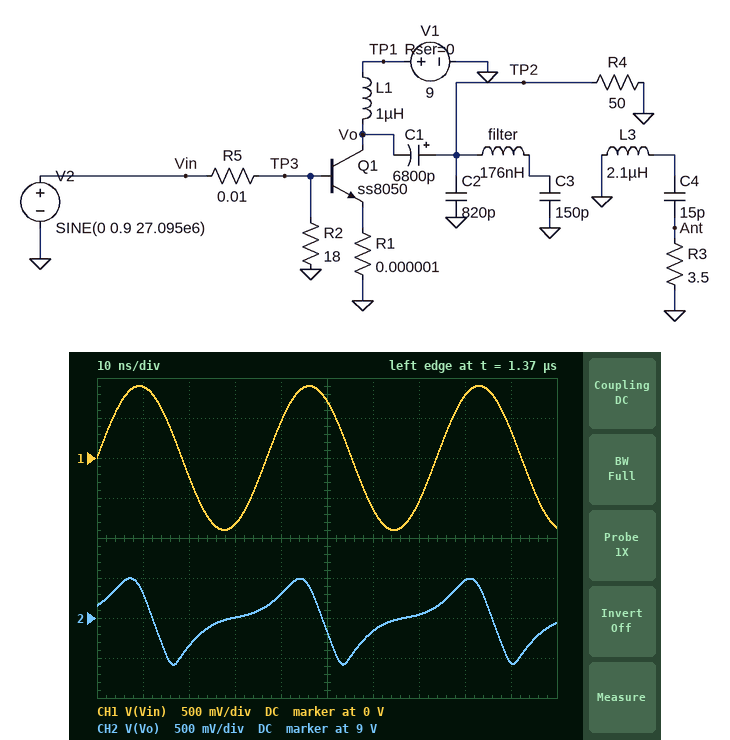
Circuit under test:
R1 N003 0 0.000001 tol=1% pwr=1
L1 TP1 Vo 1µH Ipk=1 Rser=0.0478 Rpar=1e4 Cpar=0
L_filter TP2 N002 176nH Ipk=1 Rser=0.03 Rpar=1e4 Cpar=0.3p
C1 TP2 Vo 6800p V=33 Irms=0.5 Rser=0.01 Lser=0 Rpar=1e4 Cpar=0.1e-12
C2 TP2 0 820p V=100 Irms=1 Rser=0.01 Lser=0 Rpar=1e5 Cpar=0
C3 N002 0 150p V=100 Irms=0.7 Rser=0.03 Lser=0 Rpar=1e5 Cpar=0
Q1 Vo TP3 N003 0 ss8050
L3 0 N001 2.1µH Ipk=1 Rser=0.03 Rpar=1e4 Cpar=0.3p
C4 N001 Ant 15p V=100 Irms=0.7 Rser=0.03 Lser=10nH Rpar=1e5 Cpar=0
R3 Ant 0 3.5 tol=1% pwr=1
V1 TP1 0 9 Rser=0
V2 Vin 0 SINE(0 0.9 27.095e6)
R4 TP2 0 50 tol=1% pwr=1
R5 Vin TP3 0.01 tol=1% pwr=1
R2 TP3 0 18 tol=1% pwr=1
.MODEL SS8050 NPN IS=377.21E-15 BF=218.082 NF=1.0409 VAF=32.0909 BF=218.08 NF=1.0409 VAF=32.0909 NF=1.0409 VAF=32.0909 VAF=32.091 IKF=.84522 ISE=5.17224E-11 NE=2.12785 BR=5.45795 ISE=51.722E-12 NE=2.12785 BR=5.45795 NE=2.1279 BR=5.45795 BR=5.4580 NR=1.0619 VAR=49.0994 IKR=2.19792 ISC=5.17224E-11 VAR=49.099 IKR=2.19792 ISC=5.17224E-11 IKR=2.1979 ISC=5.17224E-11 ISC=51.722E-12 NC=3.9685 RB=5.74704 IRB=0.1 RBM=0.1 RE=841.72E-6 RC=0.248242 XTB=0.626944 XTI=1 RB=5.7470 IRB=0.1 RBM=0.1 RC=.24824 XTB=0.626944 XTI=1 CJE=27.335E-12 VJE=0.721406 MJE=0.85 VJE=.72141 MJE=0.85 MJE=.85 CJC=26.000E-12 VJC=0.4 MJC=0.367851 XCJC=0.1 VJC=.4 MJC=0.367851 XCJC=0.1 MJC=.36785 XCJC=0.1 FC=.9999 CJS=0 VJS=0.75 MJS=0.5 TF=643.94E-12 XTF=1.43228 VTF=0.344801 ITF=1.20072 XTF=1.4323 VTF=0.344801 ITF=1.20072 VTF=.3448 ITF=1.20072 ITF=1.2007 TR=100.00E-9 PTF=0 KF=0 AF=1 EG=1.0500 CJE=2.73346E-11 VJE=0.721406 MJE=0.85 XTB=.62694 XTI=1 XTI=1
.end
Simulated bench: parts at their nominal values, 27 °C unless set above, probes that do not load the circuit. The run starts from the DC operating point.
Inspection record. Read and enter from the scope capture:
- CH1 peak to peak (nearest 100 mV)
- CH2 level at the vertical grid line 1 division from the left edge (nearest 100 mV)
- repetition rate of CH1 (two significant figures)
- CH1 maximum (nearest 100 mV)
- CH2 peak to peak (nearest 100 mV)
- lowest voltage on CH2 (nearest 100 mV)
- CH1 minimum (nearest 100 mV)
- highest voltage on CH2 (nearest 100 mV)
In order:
1.8 V
9.3 V
27 MHz
900 mV
1.1 V
8.4 V
-900 mV
9.5 V
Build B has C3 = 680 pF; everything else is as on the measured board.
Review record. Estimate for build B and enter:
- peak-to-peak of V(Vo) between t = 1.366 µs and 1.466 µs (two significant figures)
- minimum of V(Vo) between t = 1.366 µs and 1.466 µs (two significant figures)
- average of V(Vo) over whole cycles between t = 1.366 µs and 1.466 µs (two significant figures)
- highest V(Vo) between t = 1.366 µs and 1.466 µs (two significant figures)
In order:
1.8 V
8.0 V
9.0 V
9.8 V
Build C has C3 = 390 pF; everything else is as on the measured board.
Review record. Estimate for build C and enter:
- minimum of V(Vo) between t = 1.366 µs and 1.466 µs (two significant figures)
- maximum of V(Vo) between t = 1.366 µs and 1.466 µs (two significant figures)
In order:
7.8 V
9.9 V
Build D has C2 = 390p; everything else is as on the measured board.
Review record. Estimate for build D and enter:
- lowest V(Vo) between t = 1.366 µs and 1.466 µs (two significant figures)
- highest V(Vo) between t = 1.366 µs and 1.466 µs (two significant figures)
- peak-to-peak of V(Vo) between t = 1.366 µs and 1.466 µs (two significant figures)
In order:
8.0 V
9.9 V
1.9 V
